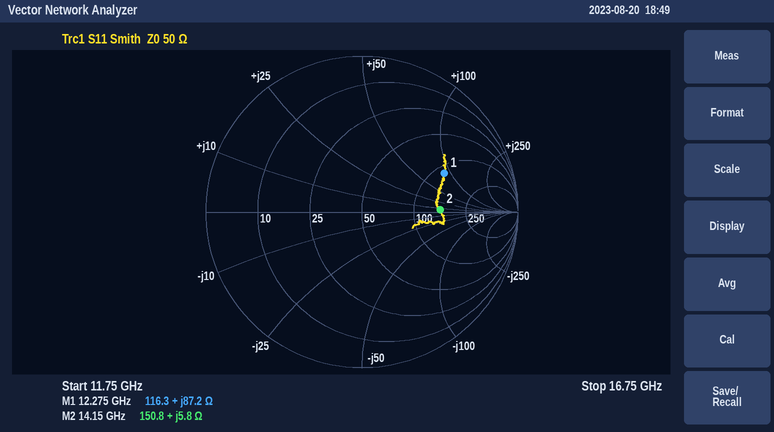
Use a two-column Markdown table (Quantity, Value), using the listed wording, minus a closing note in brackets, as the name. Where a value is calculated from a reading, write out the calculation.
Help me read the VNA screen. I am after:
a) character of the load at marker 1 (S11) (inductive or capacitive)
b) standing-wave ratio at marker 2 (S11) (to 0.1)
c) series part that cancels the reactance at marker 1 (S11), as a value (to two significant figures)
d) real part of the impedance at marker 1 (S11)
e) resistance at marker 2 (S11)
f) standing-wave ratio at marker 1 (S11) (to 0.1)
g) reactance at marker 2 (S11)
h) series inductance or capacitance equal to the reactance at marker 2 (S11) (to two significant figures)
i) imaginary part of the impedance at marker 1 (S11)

| Quantity | Value |
|---|---|
| character of the load at marker 1 (S11) | inductive |
| standing-wave ratio at marker 2 (S11) | 3.0 |
| series part that cancels the reactance at marker 1 (S11), as a value | C = 1/(2π × 12.275 GHz × 87.2 Ω) ≈ 149 fF, so 150 fF to two significant figures |
| real part of the impedance at marker 1 | 116.3 Ω |
| resistance at marker 2 | 150.8 Ω |
| standing-wave ratio at marker 1 (S11) | 3.8 |
| reactance at marker 2 | +5.8 Ω |
| series inductance or capacitance equal to the reactance at marker 2 (S11) | L = 5.8 Ω/(2π × 14.15 GHz) ≈ 65 pH |
| imaginary part of the impedance at marker 1 | +87.2 Ω |
